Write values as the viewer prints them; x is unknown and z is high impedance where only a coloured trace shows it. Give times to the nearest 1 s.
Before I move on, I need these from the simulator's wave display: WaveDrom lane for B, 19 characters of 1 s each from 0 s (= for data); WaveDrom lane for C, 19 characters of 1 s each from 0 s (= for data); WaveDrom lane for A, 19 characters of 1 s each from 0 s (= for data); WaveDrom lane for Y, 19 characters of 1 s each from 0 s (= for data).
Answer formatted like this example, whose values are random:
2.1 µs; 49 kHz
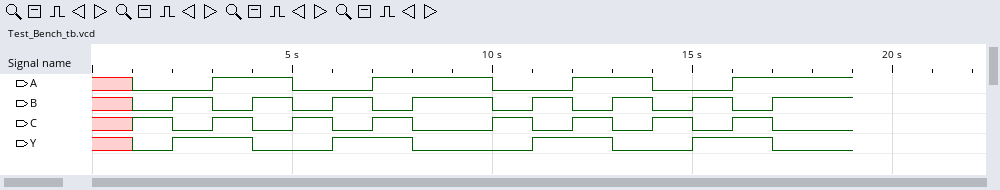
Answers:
{name: 'B', wave: 'x01010101.01010101.'}; {name: 'C', wave: 'x10101010.10101010.'}; {name: 'A', wave: 'x0.1.0.1..0.1.0.1..'}; {name: 'Y', wave: 'x01.0.1.0..1.0.1.0.'}
